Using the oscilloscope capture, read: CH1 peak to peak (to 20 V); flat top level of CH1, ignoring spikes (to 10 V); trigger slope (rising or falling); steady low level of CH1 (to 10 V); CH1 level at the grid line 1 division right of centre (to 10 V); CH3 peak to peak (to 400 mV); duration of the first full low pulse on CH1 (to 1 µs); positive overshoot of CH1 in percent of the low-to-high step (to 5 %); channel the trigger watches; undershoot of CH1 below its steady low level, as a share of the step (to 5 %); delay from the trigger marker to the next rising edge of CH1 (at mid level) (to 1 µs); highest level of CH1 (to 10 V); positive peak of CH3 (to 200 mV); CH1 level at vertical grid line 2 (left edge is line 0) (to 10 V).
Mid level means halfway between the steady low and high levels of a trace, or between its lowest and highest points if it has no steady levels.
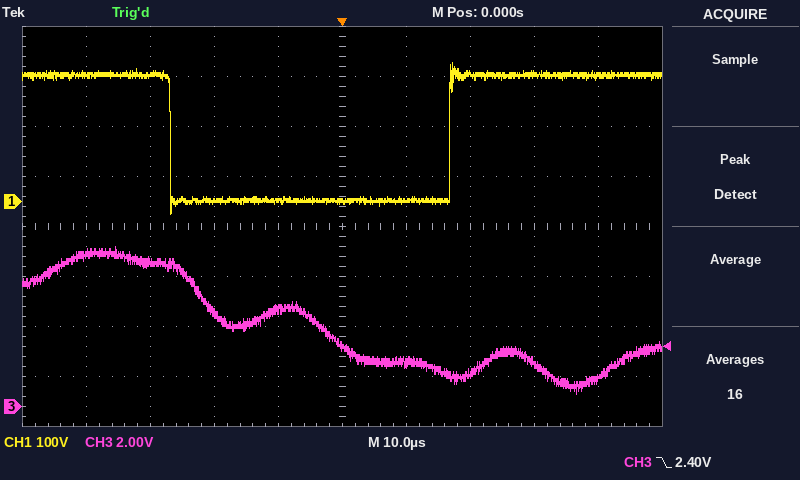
300 V
250 V
falling
0 V
0 V
6.0 V
44 µs
10 %
CH3
10 %
17 µs
280 V
6.4 V
250 V
